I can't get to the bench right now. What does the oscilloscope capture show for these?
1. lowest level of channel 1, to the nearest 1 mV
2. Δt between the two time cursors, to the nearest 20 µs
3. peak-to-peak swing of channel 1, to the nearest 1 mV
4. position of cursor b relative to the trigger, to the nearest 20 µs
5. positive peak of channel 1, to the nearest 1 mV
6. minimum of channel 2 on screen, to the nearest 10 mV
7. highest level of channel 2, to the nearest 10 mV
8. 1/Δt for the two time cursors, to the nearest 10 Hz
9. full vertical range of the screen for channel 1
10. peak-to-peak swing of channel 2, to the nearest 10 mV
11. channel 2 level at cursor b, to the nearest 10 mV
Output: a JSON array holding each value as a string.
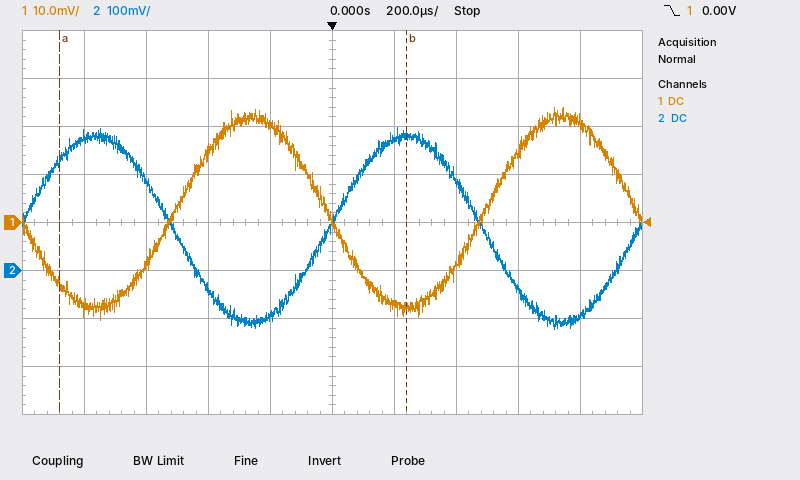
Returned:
["-20 mV", "1.12 ms", "44 mV", "+240 µs", "24 mV", "-120 mV", "300 mV", "890 Hz", "80 mV", "420 mV", "280 mV"]
